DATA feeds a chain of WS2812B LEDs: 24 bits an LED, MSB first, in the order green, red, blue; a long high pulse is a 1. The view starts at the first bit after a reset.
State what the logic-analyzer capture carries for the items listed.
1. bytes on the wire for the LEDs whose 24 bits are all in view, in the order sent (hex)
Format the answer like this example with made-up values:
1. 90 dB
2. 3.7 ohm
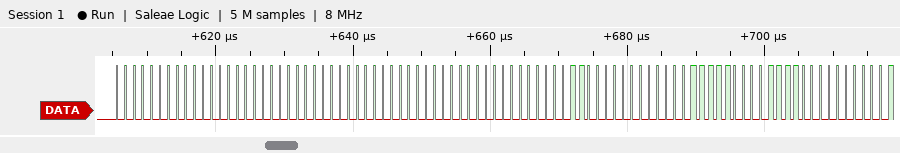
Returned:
1. 00 00 00 00 00 00 06 00 1F
